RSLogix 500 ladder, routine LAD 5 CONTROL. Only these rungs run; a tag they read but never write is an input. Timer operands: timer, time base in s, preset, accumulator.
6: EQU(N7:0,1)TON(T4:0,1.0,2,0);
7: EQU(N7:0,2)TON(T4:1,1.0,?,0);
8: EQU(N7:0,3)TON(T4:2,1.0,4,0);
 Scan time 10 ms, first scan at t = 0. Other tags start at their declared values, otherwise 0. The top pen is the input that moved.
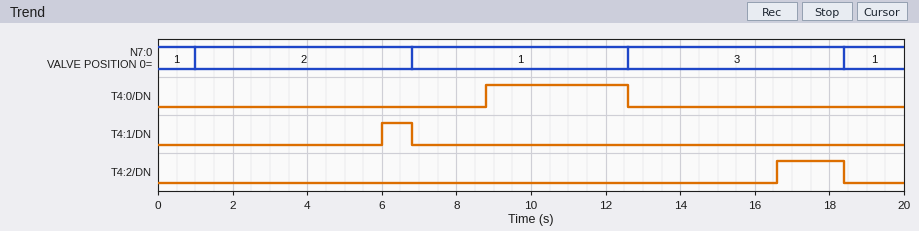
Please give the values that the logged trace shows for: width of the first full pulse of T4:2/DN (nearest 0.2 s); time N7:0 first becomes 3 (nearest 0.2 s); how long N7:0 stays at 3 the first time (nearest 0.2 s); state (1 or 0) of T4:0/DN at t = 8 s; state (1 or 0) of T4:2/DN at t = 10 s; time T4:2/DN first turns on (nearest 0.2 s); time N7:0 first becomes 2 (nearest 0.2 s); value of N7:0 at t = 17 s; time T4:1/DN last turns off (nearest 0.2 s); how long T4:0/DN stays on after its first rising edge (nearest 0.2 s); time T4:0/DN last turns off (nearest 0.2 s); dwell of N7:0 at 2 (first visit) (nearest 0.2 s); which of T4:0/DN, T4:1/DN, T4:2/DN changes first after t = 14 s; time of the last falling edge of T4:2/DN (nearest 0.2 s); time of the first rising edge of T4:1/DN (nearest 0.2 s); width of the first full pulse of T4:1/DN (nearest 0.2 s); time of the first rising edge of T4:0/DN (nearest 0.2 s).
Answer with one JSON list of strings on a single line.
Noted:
["1.8 s", "12.6 s", "5.8 s", "0", "0", "16.6 s", "1.0 s", "3", "6.8 s", "3.8 s", "12.6 s", "5.8 s", "T4:2/DN", "18.4 s", "6.0 s", "0.8 s", "8.8 s"]
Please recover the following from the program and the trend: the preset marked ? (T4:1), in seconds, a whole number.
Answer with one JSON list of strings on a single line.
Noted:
["5 s"]
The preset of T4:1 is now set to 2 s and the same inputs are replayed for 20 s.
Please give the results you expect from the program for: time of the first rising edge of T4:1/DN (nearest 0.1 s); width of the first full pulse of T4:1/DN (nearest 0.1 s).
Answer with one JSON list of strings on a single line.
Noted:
["3.0 s", "3.8 s"]
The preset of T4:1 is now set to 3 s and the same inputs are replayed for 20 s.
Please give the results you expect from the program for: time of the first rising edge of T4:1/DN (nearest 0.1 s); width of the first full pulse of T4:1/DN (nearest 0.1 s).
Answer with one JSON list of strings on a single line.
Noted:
["4.0 s", "2.8 s"]
